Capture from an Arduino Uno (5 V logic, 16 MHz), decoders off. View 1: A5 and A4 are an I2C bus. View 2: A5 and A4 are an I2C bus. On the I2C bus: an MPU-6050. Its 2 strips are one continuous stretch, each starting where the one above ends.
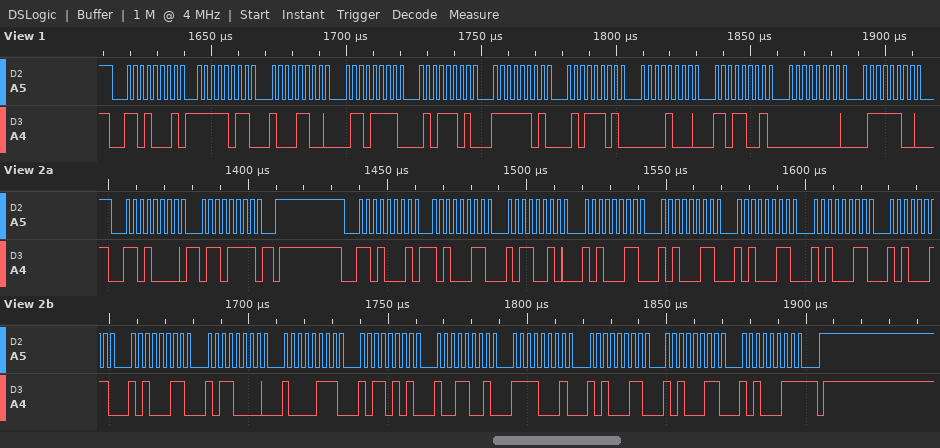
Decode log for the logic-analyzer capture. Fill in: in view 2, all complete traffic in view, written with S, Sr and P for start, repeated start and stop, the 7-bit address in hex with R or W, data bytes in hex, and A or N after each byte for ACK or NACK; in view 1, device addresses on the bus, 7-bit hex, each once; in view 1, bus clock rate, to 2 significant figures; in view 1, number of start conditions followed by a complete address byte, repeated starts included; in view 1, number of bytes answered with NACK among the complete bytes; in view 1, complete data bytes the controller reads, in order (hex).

S 68W A 6F A P S 68R A A3 A B2 A A3 A A3 A A3 A A3 A A3 A A3 A B0 A 87 A B5 A 99 A F1 A A3 A A3 A A3 N P
0x68
400 kHz
1
0
FB 8C 6F 5D FD 5D 08 D9 00 7C
